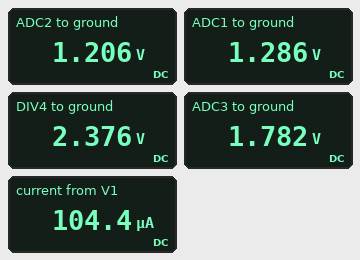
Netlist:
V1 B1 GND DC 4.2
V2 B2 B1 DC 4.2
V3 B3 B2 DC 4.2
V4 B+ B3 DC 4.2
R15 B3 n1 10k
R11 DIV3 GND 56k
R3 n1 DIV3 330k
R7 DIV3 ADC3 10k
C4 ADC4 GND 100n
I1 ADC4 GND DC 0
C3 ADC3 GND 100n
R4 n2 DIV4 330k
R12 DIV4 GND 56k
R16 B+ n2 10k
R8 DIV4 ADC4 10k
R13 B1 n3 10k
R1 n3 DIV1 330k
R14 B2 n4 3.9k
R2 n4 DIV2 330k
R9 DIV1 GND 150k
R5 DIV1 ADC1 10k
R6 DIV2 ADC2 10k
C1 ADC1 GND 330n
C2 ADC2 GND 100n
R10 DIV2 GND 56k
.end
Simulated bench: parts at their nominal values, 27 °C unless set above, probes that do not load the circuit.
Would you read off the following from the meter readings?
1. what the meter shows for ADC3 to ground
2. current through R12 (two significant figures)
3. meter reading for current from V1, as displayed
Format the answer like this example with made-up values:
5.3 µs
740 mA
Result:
1.782 V
42 µA
104.4 µA
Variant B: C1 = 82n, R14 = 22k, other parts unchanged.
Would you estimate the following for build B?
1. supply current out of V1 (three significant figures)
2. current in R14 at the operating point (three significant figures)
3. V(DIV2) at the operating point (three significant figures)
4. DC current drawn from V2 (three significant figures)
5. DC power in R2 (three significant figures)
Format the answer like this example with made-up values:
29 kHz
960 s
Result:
103 µA
20.6 µA
1.15 V
94.8 µA
140 µW
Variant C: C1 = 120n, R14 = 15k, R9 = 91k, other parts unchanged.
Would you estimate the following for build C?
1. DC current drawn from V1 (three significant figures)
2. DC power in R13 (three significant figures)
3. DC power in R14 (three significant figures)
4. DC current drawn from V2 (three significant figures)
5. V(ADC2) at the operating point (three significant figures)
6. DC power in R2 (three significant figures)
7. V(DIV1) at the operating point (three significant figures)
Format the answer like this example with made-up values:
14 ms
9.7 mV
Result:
105 µA
950 nW
6.58 µW
95.2 µA
1.17 V
145 µW
887 mV
